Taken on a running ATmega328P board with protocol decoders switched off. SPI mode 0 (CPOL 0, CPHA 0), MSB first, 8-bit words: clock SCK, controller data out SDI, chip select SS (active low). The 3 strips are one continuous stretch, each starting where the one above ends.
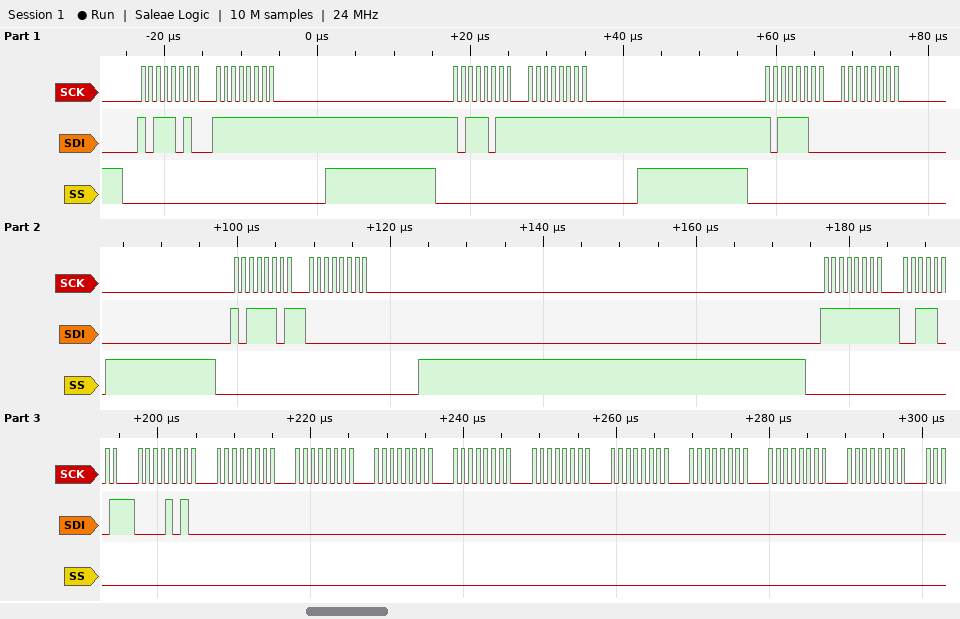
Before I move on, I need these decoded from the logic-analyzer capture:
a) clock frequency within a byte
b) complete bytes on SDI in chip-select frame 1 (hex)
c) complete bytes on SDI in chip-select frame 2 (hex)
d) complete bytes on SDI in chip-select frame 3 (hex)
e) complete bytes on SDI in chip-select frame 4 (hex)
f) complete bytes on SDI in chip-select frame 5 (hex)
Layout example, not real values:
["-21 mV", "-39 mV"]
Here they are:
["1 MHz", "BA FF", "BB FF", "BC 00", "BD 00", "FF 39 0A 00 00 00 00 00 00 00 00 00"]
